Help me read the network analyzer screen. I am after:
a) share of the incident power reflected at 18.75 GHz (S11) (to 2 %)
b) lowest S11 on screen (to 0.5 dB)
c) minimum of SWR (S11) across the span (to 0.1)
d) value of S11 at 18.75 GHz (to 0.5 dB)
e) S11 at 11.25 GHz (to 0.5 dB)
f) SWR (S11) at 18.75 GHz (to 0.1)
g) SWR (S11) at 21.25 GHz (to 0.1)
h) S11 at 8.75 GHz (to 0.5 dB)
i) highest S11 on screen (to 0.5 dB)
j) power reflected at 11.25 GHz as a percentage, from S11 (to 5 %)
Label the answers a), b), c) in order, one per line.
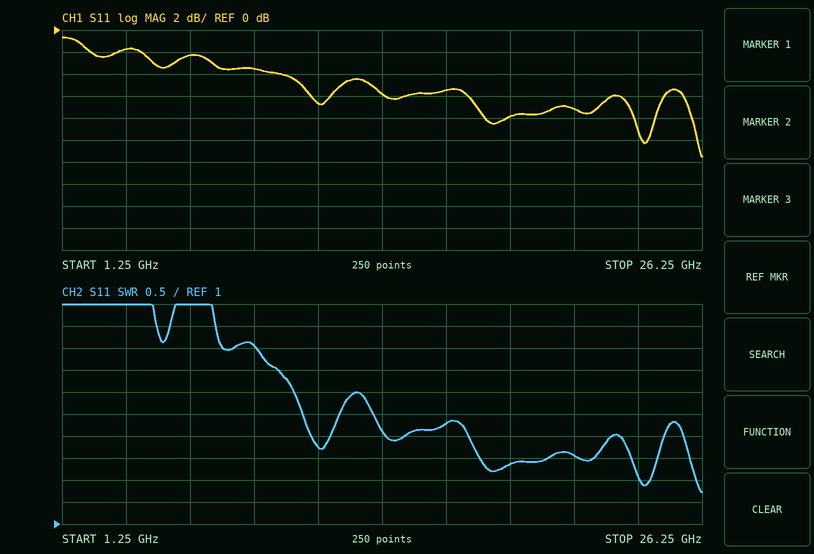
a) 16 %
b) -11.5 dB
c) 1.7
d) -8.0 dB
e) -6.5 dB
f) 2.4
g) 2.6
h) -3.5 dB
i) -0.5 dB
j) 20 %
